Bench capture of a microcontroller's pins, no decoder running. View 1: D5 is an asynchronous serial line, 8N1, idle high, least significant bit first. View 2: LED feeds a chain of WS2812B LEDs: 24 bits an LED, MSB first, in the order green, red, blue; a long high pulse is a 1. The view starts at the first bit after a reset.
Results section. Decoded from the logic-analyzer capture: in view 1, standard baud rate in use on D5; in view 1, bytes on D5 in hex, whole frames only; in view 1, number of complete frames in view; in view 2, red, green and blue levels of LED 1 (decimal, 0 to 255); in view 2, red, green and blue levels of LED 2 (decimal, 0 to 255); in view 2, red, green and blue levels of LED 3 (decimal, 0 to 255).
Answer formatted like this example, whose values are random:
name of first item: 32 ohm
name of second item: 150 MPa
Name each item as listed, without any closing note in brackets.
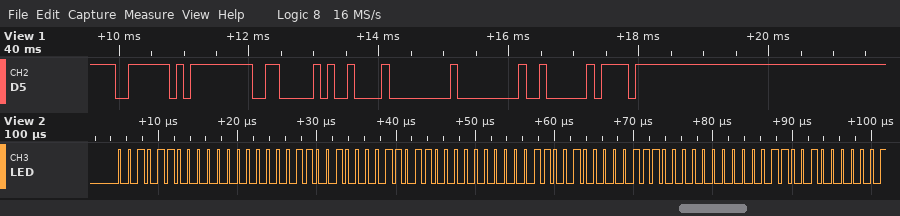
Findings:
in view 1, standard baud rate in use on D5: 9600 baud
in view 1, bytes on D5 in hex, whole frames only: 7E FF 06 09 00 00 02 EF
in view 1, number of complete frames in view: 8
in view 2, red, green and blue levels of LED 1: 0, 44, 50
in view 2, red, green and blue levels of LED 2: 0, 27, 50
in view 2, red, green and blue levels of LED 3: 0, 14, 50
